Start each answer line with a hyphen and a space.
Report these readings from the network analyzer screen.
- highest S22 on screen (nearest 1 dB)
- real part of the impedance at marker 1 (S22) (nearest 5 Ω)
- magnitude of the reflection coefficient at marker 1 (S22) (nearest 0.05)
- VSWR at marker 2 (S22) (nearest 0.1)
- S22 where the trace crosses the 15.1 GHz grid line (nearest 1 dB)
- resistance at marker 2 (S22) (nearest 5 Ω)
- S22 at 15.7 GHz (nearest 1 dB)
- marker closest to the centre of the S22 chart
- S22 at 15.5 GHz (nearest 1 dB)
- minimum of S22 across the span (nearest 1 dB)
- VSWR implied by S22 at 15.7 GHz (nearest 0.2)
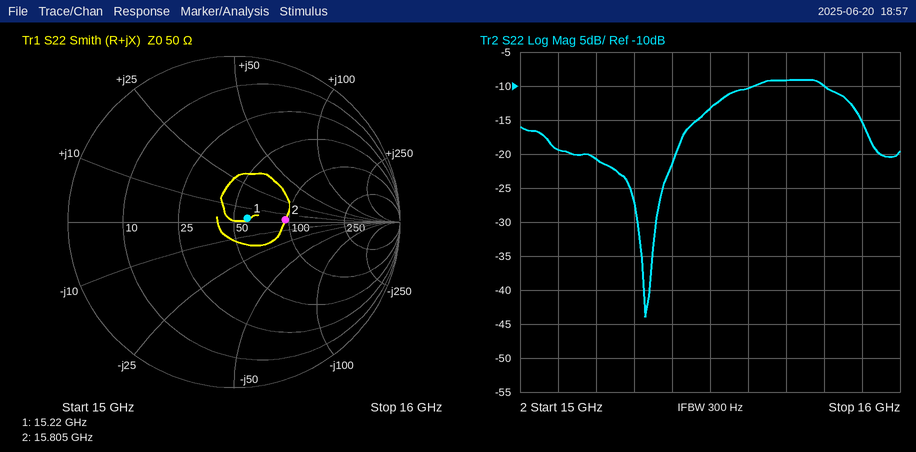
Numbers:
- -9 dB
- 60 Ω
- 0.10
- 1.9
- -19 dB
- 95 Ω
- -9 dB
- marker 1
- -13 dB
- -44 dB
- 2.0
